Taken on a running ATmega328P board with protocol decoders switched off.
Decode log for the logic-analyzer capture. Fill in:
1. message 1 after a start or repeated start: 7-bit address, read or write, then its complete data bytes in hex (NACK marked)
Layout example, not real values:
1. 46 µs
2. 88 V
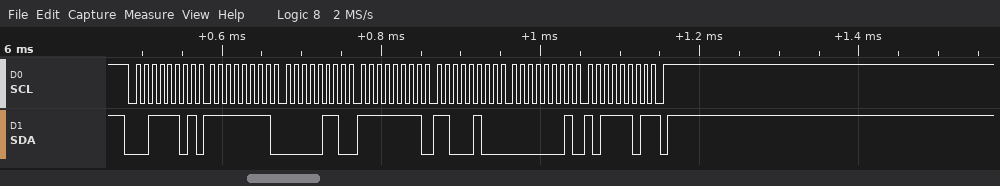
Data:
1. 0x1E read: FF 06 FF C4 01 BD NACK
